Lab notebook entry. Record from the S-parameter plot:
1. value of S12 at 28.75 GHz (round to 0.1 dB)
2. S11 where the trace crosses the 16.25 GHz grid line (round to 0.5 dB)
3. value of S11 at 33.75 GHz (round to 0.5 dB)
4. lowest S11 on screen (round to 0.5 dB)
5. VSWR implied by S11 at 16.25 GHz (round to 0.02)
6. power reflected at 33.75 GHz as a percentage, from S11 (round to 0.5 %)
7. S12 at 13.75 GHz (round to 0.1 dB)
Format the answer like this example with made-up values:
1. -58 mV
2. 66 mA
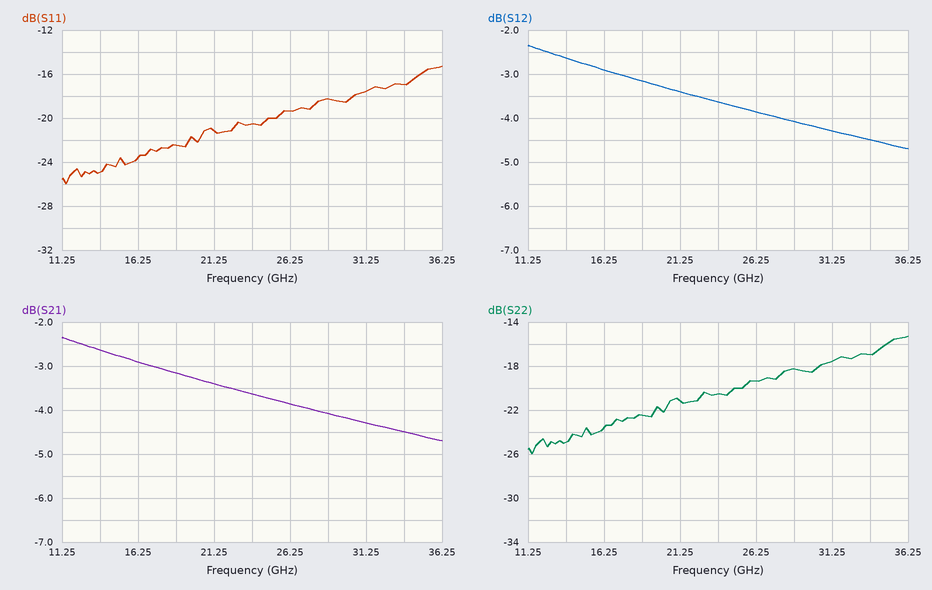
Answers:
1. -4.1 dB
2. -23.5 dB
3. -17.0 dB
4. -26.0 dB
5. 1.14
6. 2.0 %
7. -2.6 dB
